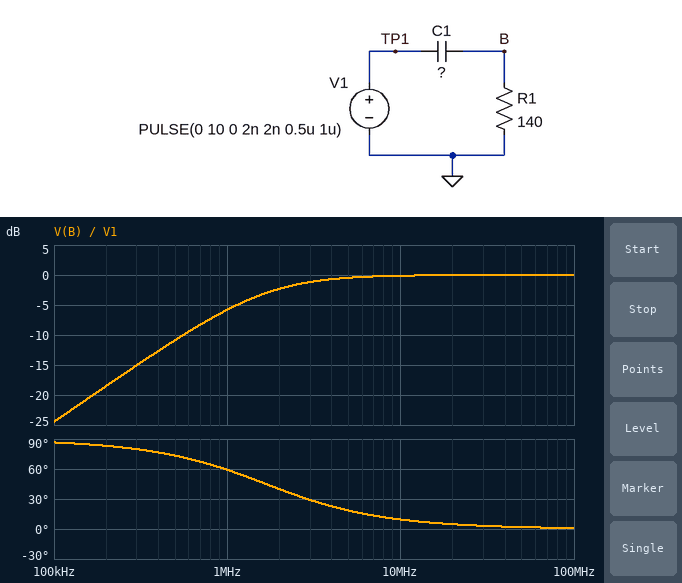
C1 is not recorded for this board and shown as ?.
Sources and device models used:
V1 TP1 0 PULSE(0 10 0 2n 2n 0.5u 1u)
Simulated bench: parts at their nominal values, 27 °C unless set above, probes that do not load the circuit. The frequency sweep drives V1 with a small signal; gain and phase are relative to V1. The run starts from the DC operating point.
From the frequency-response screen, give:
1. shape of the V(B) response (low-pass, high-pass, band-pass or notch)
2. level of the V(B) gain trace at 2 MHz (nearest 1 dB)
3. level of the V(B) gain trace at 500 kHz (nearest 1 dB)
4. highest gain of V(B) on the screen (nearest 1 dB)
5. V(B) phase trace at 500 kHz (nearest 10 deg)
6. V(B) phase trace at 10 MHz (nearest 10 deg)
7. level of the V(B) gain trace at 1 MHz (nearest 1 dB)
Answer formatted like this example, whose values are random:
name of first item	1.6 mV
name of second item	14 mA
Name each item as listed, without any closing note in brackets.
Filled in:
shape of the V(B) response	high-pass
level of the V(B) gain trace at 2 MHz	-2 dB
level of the V(B) gain trace at 500 kHz	-11 dB
highest gain of V(B) on the screen	0 dB
V(B) phase trace at 500 kHz	70 deg
V(B) phase trace at 10 MHz	10 deg
level of the V(B) gain trace at 1 MHz	-6 dB
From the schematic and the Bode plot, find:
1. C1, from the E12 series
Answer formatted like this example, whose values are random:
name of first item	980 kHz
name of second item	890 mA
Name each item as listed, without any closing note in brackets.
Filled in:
C1, from the E12 series	680 pF
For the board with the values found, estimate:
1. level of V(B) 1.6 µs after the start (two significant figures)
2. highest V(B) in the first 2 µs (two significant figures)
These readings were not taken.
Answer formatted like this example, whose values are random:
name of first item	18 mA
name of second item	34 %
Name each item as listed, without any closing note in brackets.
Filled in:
level of V(B) 1.6 µs after the start	-3.6 V
highest V(B) in the first 2 µs	9.9 V
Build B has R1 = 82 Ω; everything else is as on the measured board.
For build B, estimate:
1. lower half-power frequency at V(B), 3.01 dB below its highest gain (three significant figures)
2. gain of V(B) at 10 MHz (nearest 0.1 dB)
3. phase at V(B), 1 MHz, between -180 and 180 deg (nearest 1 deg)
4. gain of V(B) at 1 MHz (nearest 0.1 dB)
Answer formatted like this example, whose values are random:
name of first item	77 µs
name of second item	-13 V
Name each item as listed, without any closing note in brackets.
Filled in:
lower half-power frequency at V(B), 3.01 dB below its highest gain	2.85 MHz
gain of V(B) at 10 MHz	-0.3 dB
phase at V(B), 1 MHz, between -180 and 180 deg	71 deg
gain of V(B) at 1 MHz	-9.6 dB
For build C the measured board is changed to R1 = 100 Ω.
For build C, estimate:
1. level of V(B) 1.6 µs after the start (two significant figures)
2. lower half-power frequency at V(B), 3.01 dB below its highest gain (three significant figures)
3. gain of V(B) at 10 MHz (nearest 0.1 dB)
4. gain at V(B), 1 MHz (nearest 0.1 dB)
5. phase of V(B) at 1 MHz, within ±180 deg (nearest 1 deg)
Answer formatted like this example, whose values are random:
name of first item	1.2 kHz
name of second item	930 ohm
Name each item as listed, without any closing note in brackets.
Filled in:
level of V(B) 1.6 µs after the start	-2.4 V
lower half-power frequency at V(B), 3.01 dB below its highest gain	2.34 MHz
gain of V(B) at 10 MHz	-0.2 dB
gain at V(B), 1 MHz	-8.1 dB
phase of V(B) at 1 MHz, within ±180 deg	67 deg
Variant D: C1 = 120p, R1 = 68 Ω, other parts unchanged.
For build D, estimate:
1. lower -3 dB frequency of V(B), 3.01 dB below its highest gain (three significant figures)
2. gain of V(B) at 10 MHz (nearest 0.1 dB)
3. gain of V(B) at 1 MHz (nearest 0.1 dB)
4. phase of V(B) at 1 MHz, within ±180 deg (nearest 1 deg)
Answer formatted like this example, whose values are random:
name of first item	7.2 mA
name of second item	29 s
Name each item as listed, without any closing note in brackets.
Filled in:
lower -3 dB frequency of V(B), 3.01 dB below its highest gain	19.5 MHz
gain of V(B) at 10 MHz	-6.8 dB
gain of V(B) at 1 MHz	-25.8 dB
phase of V(B) at 1 MHz, within ±180 deg	87 deg
